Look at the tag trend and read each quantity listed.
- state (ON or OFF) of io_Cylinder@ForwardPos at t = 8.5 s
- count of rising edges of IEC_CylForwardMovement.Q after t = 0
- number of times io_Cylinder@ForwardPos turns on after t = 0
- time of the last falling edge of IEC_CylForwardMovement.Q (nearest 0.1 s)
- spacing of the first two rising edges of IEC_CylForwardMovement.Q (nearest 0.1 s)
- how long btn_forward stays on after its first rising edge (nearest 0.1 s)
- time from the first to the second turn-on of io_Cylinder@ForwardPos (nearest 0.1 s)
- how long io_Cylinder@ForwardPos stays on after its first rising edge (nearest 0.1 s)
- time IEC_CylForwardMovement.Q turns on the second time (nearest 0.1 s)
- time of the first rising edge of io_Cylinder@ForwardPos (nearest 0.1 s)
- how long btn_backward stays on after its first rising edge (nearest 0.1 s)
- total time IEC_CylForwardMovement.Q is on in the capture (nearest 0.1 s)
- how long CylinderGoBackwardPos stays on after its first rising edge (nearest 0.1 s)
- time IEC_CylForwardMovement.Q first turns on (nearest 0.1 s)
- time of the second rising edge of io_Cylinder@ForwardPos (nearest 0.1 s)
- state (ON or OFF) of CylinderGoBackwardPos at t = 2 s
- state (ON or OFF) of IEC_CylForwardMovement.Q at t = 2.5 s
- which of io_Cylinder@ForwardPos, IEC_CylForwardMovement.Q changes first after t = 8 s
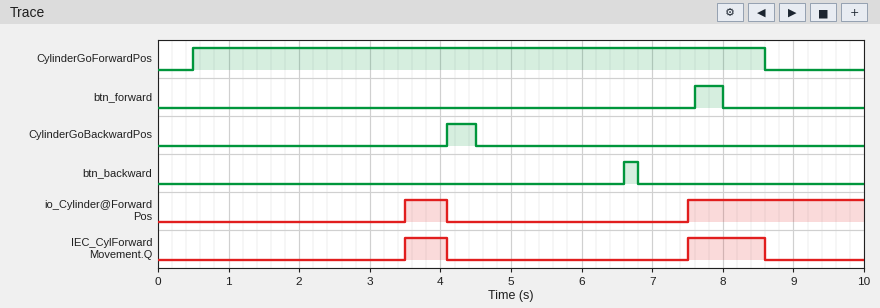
ON
2
2
8.6 s
4.0 s
0.4 s
4.0 s
0.6 s
7.5 s
3.5 s
0.2 s
1.7 s
0.4 s
3.5 s
7.5 s
OFF
OFF
IEC_CylForwardMovement.Q
